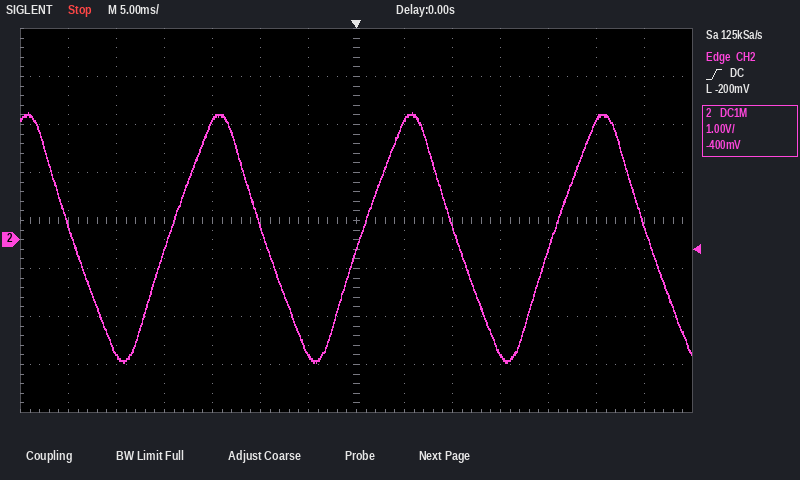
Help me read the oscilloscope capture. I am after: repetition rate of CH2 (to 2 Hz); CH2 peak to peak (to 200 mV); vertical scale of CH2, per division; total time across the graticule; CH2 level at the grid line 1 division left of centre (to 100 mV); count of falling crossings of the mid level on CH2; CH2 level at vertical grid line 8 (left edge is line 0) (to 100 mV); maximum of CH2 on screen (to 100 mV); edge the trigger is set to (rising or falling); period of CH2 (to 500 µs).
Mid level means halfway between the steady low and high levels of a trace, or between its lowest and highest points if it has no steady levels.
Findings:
50 Hz
5.2 V
1 V
70 ms
-2.4 V
4
2.5 V
2.6 V
rising
20.0 ms
